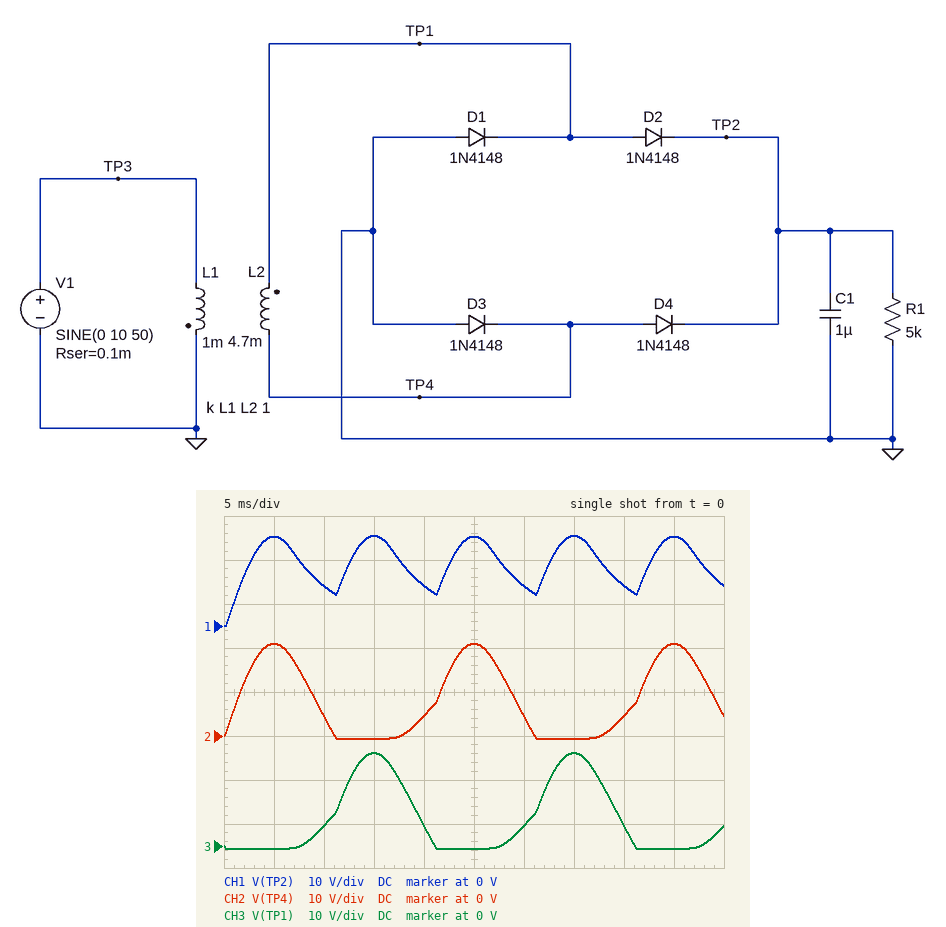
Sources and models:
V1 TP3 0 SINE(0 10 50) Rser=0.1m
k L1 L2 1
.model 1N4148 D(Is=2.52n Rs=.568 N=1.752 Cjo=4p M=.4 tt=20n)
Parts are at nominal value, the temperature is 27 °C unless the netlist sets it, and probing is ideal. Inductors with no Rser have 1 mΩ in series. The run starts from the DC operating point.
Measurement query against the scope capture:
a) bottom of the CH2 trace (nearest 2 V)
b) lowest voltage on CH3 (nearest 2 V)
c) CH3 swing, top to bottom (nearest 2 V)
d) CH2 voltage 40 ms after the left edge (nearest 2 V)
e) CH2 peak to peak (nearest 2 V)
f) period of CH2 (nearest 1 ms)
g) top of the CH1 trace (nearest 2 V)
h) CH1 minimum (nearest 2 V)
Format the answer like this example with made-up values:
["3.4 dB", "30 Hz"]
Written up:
["0 V", "0 V", "22 V", "4 V", "22 V", "20 ms", "20 V", "0 V"]
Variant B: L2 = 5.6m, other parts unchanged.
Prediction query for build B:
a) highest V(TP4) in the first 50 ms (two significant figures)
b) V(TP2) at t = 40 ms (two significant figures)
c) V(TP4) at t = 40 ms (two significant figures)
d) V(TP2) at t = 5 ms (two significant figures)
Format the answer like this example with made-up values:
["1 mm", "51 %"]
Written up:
["23 V", "10 V", "5.0 V", "22 V"]
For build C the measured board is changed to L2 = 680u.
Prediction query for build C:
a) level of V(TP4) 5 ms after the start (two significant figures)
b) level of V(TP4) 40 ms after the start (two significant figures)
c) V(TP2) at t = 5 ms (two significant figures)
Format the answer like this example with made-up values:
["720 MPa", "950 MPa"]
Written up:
["7.6 V", "1.6 V", "7.0 V"]
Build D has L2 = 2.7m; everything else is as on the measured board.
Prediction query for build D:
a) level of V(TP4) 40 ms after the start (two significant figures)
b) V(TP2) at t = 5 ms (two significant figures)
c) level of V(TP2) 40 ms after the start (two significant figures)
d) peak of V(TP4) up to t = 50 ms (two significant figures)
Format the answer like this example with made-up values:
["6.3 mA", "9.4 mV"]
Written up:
["3.4 V", "15 V", "6.8 V", "16 V"]
